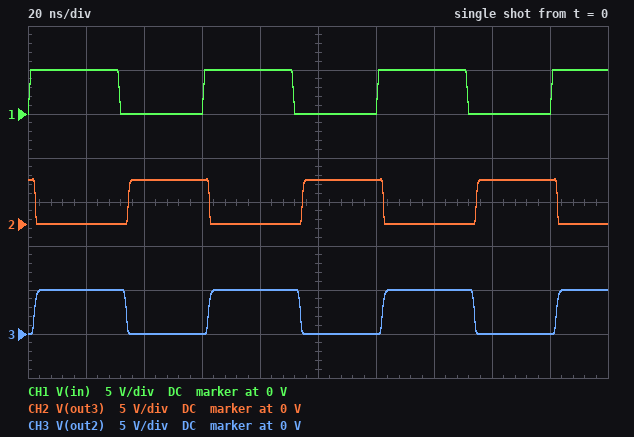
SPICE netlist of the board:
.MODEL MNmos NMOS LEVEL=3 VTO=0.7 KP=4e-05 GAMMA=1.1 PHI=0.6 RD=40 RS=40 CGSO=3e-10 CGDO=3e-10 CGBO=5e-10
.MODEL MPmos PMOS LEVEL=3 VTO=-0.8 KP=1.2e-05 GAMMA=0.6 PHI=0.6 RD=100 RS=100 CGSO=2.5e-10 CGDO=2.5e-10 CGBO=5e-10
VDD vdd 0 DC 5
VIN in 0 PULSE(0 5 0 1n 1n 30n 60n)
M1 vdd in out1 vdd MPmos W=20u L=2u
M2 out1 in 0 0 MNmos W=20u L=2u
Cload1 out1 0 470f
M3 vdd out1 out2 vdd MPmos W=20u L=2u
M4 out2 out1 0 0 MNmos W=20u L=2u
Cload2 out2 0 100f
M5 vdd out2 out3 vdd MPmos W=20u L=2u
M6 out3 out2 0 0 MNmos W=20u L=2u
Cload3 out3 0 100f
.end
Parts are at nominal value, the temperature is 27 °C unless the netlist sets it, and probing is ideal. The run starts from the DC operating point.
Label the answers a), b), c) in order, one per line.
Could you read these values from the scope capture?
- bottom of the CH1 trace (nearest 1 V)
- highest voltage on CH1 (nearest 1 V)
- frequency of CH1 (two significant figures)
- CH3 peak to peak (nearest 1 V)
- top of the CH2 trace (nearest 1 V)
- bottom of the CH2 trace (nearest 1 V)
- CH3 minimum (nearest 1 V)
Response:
a) 0 V
b) 5 V
c) 17 MHz
d) 5 V
e) 5 V
f) 0 V
g) 0 V
